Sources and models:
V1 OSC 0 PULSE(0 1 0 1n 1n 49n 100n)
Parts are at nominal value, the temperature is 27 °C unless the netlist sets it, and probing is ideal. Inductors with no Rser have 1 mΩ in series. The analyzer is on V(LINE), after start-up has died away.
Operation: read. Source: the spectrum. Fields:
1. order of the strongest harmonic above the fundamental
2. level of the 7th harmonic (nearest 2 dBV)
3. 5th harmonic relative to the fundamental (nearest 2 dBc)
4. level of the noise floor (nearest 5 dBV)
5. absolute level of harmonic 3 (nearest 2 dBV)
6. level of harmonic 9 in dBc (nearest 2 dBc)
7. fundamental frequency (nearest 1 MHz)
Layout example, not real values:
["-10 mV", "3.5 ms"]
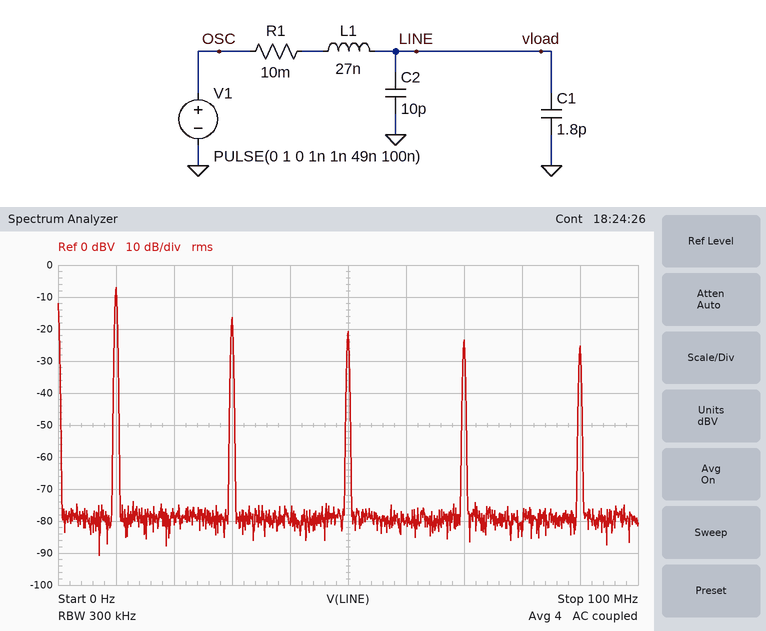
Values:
["3", "-24 dBV", "-14 dBc", "-80 dBV", "-16 dBV", "-18 dBc", "10 MHz"]
